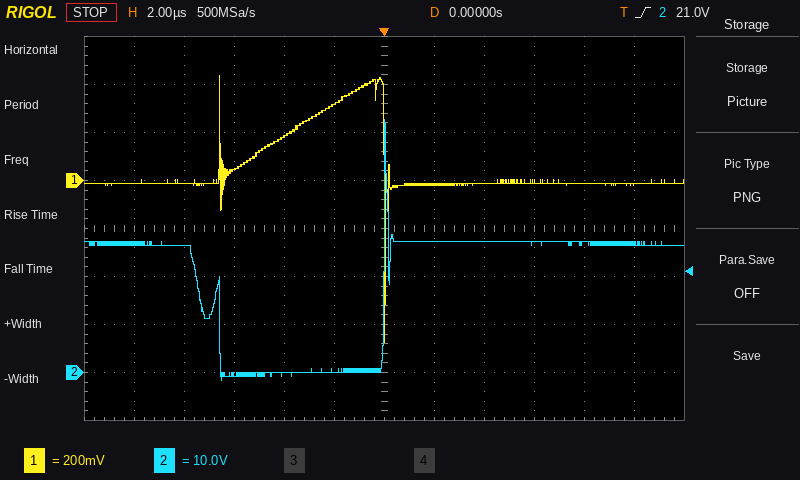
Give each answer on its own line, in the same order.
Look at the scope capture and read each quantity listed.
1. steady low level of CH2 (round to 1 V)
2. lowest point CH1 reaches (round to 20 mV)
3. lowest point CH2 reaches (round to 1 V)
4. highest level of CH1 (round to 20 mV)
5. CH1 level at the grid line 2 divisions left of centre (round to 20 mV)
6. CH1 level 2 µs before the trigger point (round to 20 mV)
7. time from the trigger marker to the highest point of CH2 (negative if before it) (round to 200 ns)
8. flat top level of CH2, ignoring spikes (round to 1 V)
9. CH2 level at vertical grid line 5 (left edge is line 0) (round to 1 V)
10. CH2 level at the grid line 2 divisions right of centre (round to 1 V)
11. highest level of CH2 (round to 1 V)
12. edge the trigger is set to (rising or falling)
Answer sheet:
0 V
-680 mV
-2 V
440 mV
180 mV
320 mV
0.0 µs
27 V
0 V
27 V
53 V
rising
